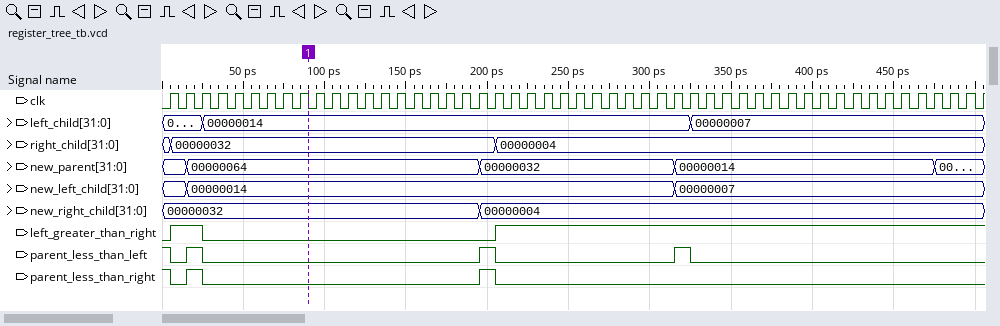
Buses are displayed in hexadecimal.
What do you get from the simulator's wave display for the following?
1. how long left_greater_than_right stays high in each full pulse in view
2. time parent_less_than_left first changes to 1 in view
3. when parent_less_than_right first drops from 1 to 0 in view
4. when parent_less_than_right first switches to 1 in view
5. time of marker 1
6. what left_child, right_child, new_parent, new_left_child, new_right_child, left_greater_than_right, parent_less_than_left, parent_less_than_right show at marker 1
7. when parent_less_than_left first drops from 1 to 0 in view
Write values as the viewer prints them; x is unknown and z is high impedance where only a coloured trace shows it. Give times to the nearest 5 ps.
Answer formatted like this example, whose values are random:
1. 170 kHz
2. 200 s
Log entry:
1. 20 ps
2. 15 ps
3. 5 ps
4. 15 ps
5. 90 ps
6. left_child=00000014, right_child=00000032, new_parent=00000064, new_left_child=00000014, new_right_child=00000032, left_greater_than_right=0, parent_less_than_left=0, parent_less_than_right=0
7. 5 ps
